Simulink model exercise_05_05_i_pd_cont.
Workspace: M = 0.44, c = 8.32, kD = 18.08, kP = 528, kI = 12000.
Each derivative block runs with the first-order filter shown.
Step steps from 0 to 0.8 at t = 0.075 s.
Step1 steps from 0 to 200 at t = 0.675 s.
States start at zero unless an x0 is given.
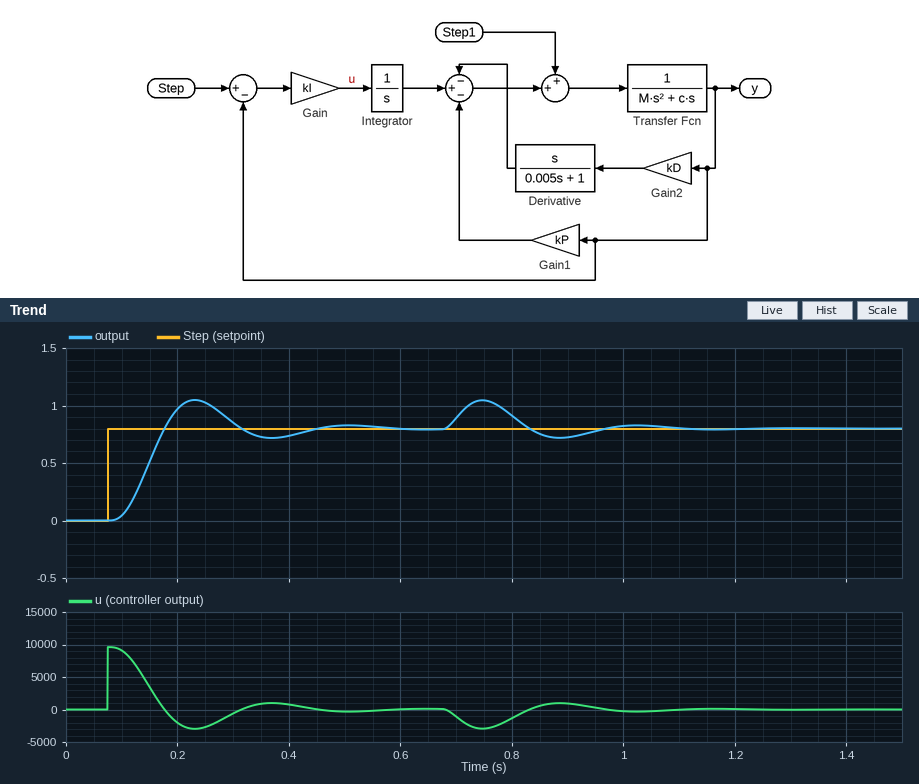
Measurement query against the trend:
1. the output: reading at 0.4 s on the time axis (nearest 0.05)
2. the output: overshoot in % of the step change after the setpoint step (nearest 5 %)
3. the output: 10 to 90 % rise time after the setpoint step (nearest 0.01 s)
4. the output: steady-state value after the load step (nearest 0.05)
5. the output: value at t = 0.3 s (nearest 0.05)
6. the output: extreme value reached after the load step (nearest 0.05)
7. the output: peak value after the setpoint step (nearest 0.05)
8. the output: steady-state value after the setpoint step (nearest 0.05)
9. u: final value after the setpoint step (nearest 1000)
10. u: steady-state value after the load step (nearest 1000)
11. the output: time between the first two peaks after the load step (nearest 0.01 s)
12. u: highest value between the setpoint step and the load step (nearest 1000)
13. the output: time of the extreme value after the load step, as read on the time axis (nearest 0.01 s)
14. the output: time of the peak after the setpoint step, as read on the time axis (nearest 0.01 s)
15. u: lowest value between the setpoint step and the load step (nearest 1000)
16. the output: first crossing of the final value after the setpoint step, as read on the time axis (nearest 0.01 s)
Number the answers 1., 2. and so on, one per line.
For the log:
1. 0.75
2. 30 %
3. 0.06 s
4. 0.80
5. 0.85
6. 1.05
7. 1.05
8. 0.80
9. 0
10. 0
11. 0.28 s
12. 10000
13. 0.75 s
14. 0.23 s
15. -3000
16. 0.18 s
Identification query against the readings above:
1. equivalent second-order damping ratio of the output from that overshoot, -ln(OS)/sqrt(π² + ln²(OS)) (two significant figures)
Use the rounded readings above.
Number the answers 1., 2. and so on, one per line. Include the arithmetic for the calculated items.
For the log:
1. ln(0.3) = -1.204; 1.204 / sqrt(9.870 + 1.450) = 0.36
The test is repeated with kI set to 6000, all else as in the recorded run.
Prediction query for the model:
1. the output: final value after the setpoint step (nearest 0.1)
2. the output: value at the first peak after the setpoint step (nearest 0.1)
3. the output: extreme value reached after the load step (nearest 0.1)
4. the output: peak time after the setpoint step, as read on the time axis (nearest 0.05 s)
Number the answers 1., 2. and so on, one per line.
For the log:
1. 0.8
2. 0.9
3. 1.1
4. 0.30 s
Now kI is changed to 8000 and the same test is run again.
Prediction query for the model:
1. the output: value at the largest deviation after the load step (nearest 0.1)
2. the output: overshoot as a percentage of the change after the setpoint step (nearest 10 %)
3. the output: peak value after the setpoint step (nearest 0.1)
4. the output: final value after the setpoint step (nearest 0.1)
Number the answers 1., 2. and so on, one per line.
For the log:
1. 1.1
2. 20 %
3. 0.9
4. 0.8
